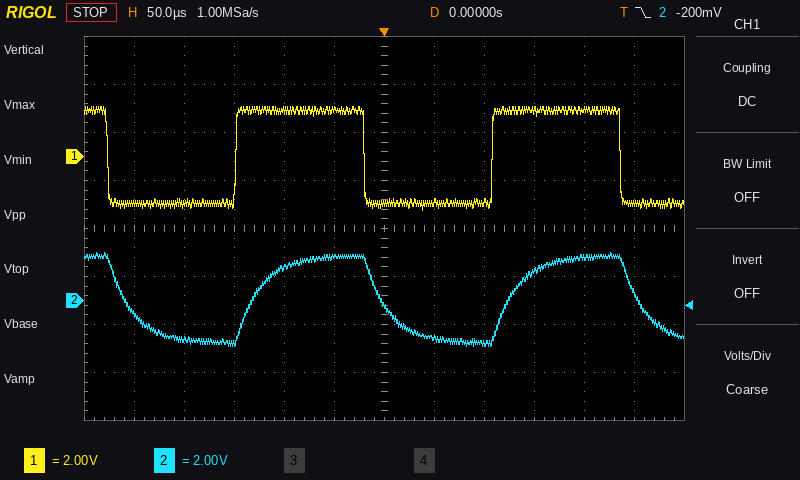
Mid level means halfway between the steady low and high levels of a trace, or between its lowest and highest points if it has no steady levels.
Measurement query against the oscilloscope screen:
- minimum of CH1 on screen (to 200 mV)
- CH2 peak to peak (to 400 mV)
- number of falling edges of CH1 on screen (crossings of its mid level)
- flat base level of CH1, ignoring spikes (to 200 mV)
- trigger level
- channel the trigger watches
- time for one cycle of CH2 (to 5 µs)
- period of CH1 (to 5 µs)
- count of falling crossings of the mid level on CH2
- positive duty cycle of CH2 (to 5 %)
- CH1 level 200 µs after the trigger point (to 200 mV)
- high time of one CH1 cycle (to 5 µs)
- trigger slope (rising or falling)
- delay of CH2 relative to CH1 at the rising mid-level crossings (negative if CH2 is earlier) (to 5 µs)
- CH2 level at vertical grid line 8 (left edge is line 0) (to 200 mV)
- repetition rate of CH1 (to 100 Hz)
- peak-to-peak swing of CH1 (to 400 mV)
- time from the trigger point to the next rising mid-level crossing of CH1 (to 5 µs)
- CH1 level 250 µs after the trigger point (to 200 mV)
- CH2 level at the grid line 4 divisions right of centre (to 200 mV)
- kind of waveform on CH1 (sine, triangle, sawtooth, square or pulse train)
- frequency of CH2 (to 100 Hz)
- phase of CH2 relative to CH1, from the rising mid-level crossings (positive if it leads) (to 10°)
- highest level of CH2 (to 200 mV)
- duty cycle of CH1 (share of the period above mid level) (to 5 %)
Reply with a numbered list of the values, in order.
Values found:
1. -2.2 V
2. 4.0 V
3. 3
4. -2.0 V
5. -200 mV
6. CH2
7. 255 µs
8. 255 µs
9. 3
10. 50 %
11. 2.0 V
12. 130 µs
13. falling
14. +15 µs
15. -1.8 V
16. 3.9 kHz
17. 4.4 V
18. 110 µs
19. -2.0 V
20. 1.8 V
21. square
22. 3.9 kHz
23. -20°
24. 2.0 V
25. 50 %
